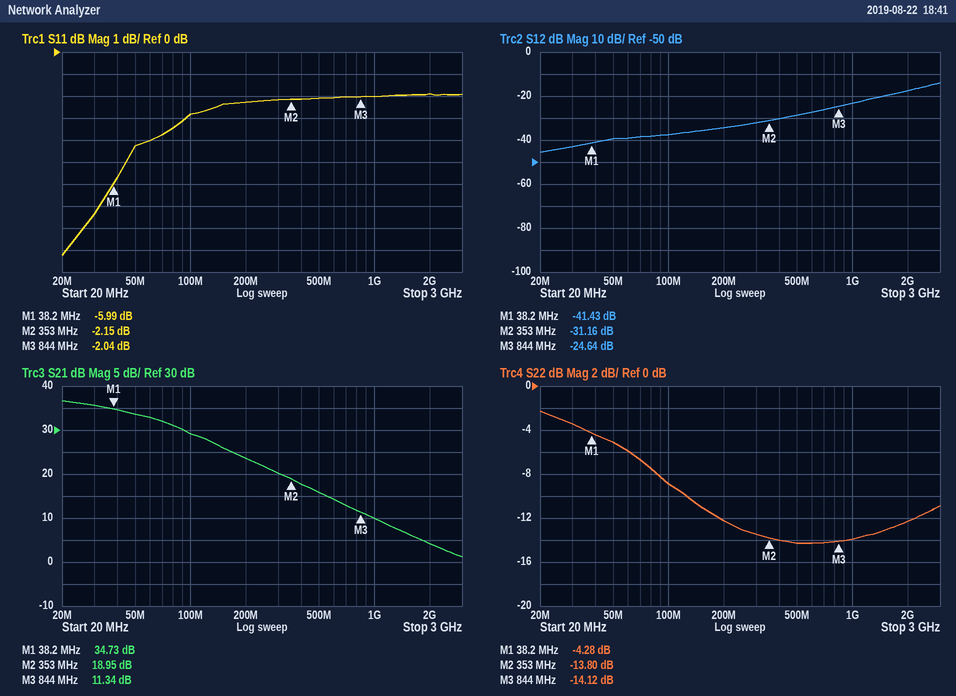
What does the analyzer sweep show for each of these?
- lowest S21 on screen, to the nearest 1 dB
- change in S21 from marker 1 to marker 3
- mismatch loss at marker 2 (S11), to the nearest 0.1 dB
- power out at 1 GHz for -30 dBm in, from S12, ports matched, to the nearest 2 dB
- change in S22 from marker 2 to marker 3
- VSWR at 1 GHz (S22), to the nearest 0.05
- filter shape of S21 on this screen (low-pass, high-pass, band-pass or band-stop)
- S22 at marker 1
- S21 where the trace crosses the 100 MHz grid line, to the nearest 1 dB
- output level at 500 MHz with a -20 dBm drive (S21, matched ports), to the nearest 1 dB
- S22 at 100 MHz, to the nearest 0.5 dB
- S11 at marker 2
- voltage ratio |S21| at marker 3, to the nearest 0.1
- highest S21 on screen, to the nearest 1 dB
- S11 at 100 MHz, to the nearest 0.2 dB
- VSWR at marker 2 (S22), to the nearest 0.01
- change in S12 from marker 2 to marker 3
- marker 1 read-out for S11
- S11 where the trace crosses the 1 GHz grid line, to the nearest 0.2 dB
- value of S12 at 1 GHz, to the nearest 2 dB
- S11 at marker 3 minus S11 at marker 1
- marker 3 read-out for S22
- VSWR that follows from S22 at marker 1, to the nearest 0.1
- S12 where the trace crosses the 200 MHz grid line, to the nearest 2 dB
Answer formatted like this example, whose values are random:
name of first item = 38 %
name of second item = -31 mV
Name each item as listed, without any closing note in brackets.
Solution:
lowest S21 on screen, to the nearest 1 dB = 1 dB
change in S21 from marker 1 to marker 3 = -23.39 dB
mismatch loss at marker 2 (S11), to the nearest 0.1 dB = 4.1 dB
power out at 1 GHz for -30 dBm in, from S12, ports matched, to the nearest 2 dB = -54 dBm
change in S22 from marker 2 to marker 3 = -0.32 dB
VSWR at 1 GHz (S22), to the nearest 0.05 = 1.50
filter shape of S21 on this screen = low-pass
S22 at marker 1 = -4.28 dB
S21 where the trace crosses the 100 MHz grid line, to the nearest 1 dB = 29 dB
output level at 500 MHz with a -20 dBm drive (S21, matched ports), to the nearest 1 dB = -4 dBm
S22 at 100 MHz, to the nearest 0.5 dB = -9.0 dB
S11 at marker 2 = -2.15 dB
voltage ratio |S21| at marker 3, to the nearest 0.1 = 3.7
highest S21 on screen, to the nearest 1 dB = 37 dB
S11 at 100 MHz, to the nearest 0.2 dB = -2.8 dB
VSWR at marker 2 (S22), to the nearest 0.01 = 1.51
change in S12 from marker 2 to marker 3 = 6.52 dB
marker 1 read-out for S11 = -5.99 dB
S11 where the trace crosses the 1 GHz grid line, to the nearest 0.2 dB = -2.0 dB
value of S12 at 1 GHz, to the nearest 2 dB = -24 dB
S11 at marker 3 minus S11 at marker 1 = 3.95 dB
marker 3 read-out for S22 = -14.12 dB
VSWR that follows from S22 at marker 1, to the nearest 0.1 = 4.1
S12 where the trace crosses the 200 MHz grid line, to the nearest 2 dB = -34 dB
